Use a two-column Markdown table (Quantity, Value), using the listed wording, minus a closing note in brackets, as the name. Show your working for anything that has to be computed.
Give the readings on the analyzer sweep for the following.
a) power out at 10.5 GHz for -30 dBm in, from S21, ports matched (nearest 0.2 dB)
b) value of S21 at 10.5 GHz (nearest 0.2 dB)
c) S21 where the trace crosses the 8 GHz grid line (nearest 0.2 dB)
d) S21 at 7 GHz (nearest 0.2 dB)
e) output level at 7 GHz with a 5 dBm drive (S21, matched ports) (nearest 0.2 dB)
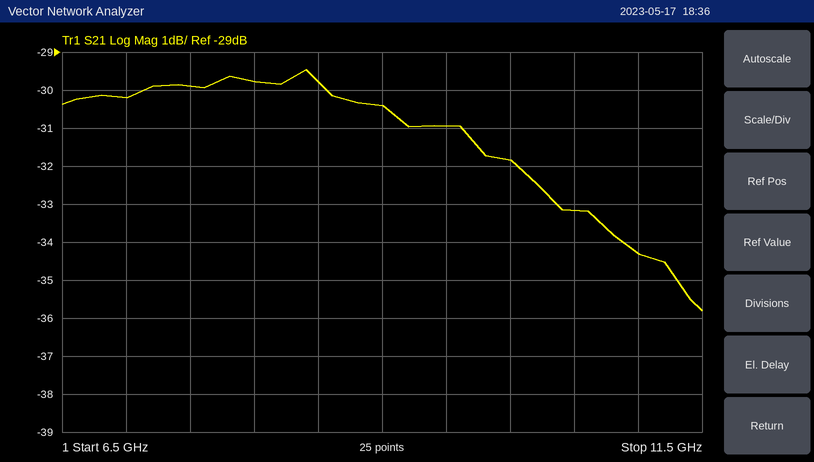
| Quantity | Value |
|---|---|
| power out at 10.5 GHz for -30 dBm in, from S21, ports matched | -30 dBm + (-33.2 dB) = -63.2 dBm |
| value of S21 at 10.5 GHz | -33.2 dB |
| S21 where the trace crosses the 8 GHz grid line | -29.8 dB |
| S21 at 7 GHz | -30.2 dB |
| output level at 7 GHz with a 5 dBm drive (S21, matched ports) | 5 dBm + (-30.2 dB) = -25.2 dBm |
